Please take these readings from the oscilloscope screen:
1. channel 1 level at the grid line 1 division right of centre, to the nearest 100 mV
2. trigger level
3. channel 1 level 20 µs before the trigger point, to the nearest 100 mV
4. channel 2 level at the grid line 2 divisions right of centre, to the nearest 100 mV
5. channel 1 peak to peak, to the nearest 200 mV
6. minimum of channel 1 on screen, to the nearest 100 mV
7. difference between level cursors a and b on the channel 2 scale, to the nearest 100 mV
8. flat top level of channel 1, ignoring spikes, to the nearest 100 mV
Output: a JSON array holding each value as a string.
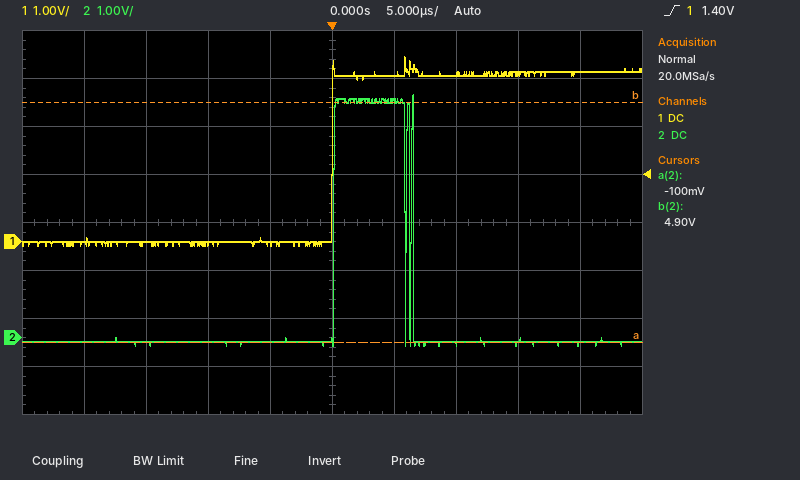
["3.5 V", "1.40 V", "0.0 V", "-100 mV", "4.0 V", "-100 mV", "5.0 V", "3.5 V"]
